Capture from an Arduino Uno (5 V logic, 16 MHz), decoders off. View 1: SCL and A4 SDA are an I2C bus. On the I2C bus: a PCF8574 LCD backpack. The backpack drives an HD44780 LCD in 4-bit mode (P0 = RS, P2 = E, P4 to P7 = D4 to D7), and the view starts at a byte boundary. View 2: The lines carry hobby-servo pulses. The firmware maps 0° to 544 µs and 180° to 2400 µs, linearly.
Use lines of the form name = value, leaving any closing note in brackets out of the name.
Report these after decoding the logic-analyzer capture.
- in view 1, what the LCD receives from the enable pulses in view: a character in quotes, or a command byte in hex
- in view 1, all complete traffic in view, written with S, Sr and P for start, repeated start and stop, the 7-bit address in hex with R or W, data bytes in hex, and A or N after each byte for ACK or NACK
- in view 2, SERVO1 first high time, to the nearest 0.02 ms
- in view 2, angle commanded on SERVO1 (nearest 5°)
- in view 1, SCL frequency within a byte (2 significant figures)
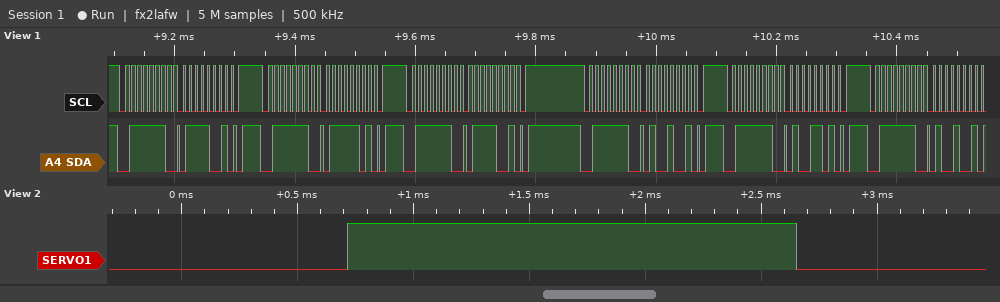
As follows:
in view 1, what the LCD receives from the enable pulses in view: a character in quotes, or a command byte in hex = 't'
in view 1, all complete traffic in view, written with S, Sr and P for start, repeated start and stop, the 7-bit address in hex with R or W, data bytes in hex, and A or N after each byte for ACK or NACK = S 3FW A 79 A P S 3FW A 7D A P S 3FW A 79 A P S 3FW A 49 A P S 3FW A 4D A P S 3FW A 49 A
in view 2, SERVO1 first high time, to the nearest 0.02 ms = 1.94 ms
in view 2, angle commanded on SERVO1 = 135°
in view 1, SCL frequency within a byte = 100 kHz
